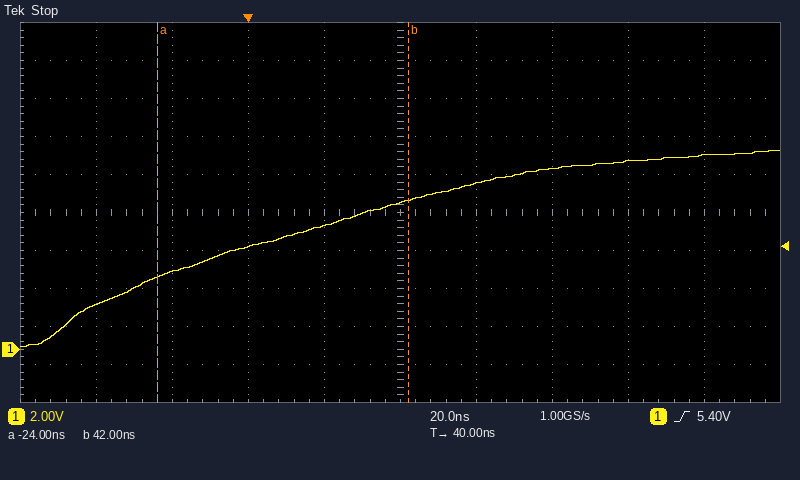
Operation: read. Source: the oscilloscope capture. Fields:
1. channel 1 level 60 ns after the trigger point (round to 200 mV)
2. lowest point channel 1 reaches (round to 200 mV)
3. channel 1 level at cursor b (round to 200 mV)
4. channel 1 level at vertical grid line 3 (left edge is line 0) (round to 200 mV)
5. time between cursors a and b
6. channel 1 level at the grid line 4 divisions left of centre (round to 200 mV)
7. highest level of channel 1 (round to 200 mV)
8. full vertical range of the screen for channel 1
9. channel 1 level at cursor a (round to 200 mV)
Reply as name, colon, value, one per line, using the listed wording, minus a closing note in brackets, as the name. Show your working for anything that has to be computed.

channel 1 level 60 ns after the trigger point: 8.8 V
lowest point channel 1 reaches: 200 mV
channel 1 level at cursor b: 7.8 V
channel 1 level at vertical grid line 3 (left edge is line 0): 5.4 V
time between cursors a and b: 42 ns − (-24 ns) = 66 ns
channel 1 level at the grid line 4 divisions left of centre: 2.4 V
highest level of channel 1: 10.4 V
full vertical range of the screen for channel 1: 20 V
channel 1 level at cursor a: 3.8 V
